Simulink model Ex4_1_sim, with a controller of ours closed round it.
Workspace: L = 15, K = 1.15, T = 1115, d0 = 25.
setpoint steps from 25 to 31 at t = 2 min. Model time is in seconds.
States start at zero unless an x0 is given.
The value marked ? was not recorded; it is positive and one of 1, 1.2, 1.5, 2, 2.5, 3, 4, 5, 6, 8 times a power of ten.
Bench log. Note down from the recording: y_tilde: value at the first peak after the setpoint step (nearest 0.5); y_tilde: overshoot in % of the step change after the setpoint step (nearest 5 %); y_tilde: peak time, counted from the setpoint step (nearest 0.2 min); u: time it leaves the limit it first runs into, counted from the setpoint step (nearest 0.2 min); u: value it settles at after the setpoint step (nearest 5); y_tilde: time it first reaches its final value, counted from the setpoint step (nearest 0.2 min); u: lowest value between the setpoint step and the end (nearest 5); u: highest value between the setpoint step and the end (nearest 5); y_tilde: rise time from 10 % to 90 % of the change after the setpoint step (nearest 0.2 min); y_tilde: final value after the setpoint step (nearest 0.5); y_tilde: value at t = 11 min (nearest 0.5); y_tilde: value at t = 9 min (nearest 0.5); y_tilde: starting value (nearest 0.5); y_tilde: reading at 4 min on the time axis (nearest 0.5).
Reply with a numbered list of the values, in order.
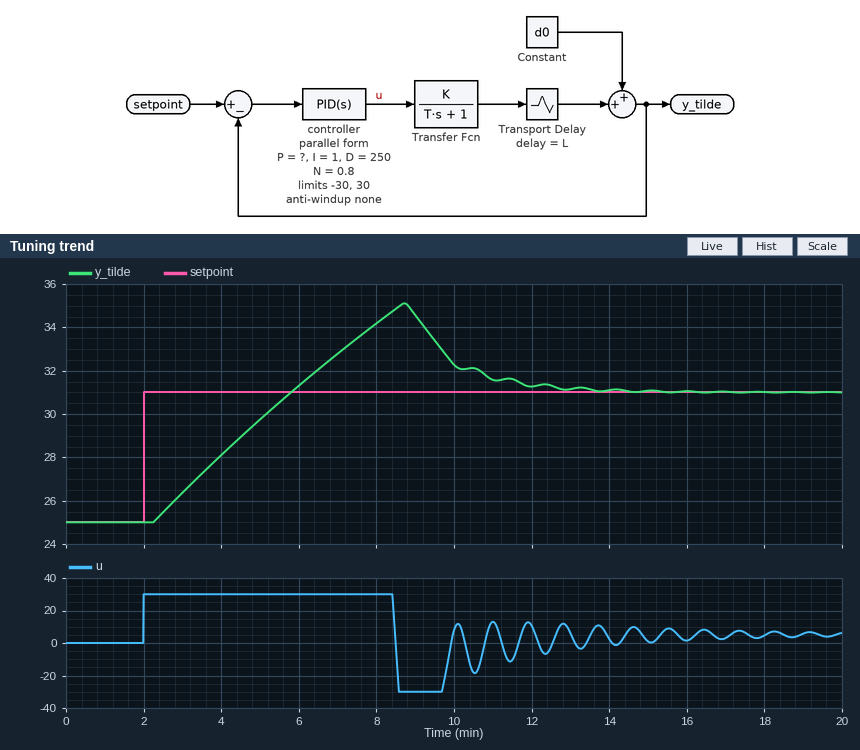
1. 35.0
2. 70 %
3. 6.8 min
4. 6.4 min
5. 5
6. 3.8 min
7. -30
8. 30
9. 2.8 min
10. 31.0
11. 31.5
12. 34.5
13. 25.0
14. 28.0
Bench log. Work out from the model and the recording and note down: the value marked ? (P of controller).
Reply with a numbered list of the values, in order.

1. 100
